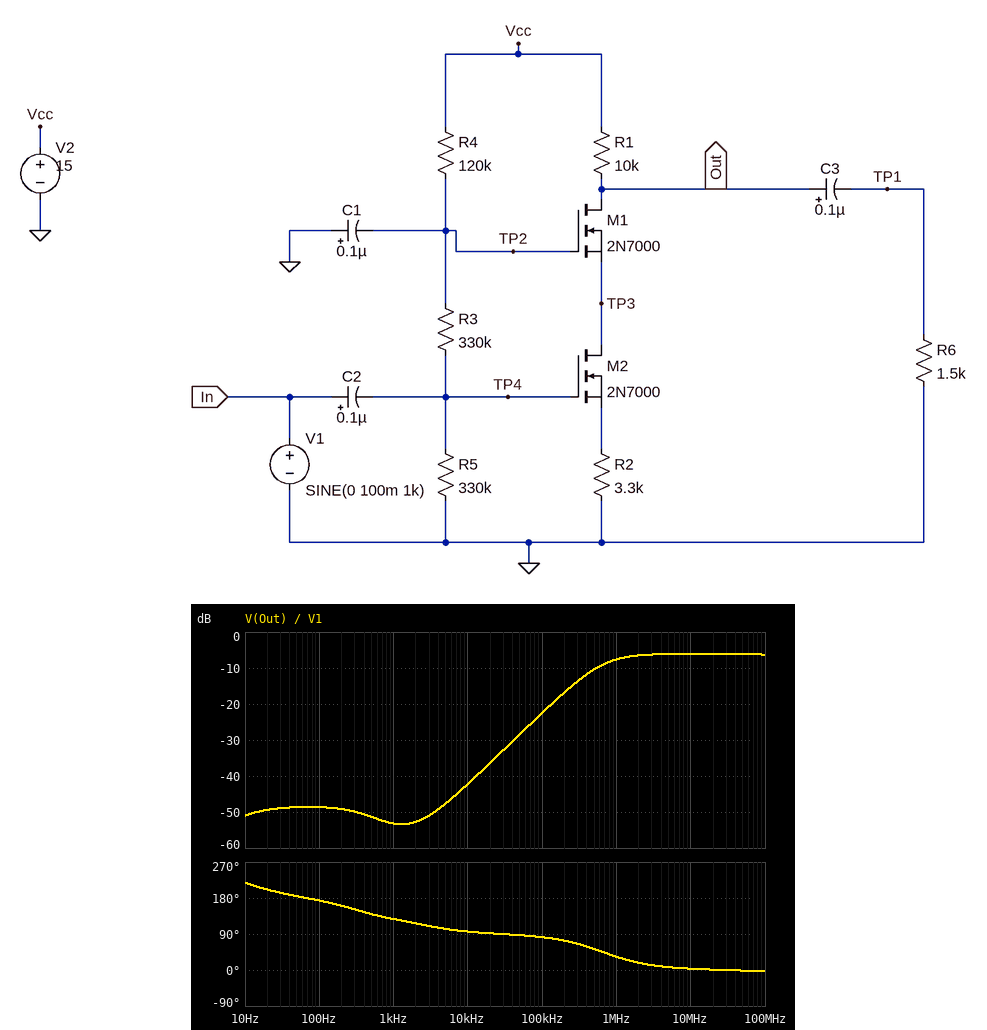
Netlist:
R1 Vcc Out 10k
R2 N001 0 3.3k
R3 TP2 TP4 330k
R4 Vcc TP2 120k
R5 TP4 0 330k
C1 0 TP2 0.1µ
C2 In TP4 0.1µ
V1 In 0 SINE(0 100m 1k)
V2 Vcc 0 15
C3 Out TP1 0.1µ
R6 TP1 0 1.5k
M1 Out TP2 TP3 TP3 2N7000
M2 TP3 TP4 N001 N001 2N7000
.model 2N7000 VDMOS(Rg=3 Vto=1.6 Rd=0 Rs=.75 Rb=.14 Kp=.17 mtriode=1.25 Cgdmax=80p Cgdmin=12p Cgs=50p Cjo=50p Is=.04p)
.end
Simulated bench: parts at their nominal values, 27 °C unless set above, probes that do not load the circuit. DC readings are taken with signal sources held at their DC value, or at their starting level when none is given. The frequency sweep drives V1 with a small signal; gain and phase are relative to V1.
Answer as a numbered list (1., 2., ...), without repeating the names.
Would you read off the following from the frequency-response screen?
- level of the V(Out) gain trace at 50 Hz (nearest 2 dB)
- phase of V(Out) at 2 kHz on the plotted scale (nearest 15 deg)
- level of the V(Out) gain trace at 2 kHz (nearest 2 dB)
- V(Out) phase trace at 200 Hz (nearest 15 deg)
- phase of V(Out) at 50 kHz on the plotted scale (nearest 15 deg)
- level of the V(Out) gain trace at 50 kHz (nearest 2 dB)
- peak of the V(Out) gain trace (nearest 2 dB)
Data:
1. -48 dB
2. 120 deg
3. -52 dB
4. 165 deg
5. 90 deg
6. -28 dB
7. -6 dB
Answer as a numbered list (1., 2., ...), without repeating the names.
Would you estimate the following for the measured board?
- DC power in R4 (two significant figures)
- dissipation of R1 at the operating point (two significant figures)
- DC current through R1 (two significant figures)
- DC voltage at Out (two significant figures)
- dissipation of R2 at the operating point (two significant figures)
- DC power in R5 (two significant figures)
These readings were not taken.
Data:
1. 44 µW
2. 13 mW
3. 1.1 mA
4. 3.7 V
5. 4.2 mW
6. 120 µW
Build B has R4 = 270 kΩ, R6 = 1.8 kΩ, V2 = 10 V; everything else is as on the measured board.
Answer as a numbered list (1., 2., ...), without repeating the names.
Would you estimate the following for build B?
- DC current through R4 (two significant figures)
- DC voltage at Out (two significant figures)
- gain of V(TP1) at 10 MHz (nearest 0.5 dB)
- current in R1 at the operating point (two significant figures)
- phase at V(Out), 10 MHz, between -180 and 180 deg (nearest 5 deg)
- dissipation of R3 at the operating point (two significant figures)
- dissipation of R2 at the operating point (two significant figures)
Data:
1. 11 µA
2. 4.2 V
3. -11.5 dB
4. 580 µA
5. 15 deg
6. 38 µW
7. 1.1 mW
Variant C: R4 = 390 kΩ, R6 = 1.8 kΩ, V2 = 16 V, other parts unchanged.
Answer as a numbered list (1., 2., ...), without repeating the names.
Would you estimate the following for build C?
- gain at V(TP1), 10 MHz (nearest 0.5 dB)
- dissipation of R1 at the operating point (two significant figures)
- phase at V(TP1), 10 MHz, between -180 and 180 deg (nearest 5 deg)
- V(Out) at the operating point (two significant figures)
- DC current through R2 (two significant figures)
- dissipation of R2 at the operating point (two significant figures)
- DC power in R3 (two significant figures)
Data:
1. -12.5 dB
2. 10 mW
3. 15 deg
4. 5.8 V
5. 1.0 mA
6. 3.4 mW
7. 77 µW
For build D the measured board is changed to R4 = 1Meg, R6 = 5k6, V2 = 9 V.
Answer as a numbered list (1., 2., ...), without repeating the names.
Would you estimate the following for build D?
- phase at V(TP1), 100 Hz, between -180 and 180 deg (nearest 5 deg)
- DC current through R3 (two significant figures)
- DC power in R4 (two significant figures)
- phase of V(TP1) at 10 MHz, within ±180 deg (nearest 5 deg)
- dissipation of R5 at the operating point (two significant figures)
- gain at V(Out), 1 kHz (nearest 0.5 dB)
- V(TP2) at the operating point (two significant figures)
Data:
1. -130 deg
2. 5.4 µA
3. 29 µW
4. -35 deg
5. 9.7 µW
6. -0.5 dB
7. 3.6 V
